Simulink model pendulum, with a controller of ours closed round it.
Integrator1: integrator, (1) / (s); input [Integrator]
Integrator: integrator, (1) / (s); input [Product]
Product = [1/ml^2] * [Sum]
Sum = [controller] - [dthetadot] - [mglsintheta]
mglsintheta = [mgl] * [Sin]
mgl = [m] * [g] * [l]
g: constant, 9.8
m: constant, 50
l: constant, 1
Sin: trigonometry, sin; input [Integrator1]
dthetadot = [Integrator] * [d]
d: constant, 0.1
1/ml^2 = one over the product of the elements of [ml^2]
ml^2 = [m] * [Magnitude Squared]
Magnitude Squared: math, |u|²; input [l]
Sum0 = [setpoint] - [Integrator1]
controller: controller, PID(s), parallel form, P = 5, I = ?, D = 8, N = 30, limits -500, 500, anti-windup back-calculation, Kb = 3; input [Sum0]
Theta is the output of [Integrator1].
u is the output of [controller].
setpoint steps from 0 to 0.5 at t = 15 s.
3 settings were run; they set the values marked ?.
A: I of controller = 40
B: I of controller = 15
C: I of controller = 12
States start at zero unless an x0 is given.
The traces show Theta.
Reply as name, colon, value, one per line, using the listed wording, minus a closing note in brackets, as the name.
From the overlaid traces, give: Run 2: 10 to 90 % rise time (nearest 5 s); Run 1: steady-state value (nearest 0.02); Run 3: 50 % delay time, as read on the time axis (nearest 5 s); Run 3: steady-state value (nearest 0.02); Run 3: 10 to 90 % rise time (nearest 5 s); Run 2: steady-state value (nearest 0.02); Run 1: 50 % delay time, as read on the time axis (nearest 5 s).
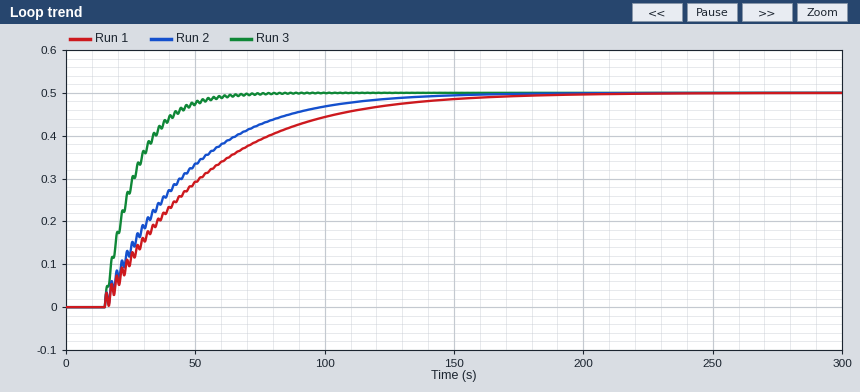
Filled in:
Run 2: 10 to 90 % rise time: 70 s
Run 1: steady-state value: 0.50
Run 3: 50 % delay time, as read on the time axis: 25 s
Run 3: steady-state value: 0.50
Run 3: 10 to 90 % rise time: 25 s
Run 2: steady-state value: 0.50
Run 1: 50 % delay time, as read on the time axis: 45 s
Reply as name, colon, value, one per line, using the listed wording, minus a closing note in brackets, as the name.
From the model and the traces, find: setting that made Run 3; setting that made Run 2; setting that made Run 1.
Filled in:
setting that made Run 3: A
setting that made Run 2: B
setting that made Run 1: C
